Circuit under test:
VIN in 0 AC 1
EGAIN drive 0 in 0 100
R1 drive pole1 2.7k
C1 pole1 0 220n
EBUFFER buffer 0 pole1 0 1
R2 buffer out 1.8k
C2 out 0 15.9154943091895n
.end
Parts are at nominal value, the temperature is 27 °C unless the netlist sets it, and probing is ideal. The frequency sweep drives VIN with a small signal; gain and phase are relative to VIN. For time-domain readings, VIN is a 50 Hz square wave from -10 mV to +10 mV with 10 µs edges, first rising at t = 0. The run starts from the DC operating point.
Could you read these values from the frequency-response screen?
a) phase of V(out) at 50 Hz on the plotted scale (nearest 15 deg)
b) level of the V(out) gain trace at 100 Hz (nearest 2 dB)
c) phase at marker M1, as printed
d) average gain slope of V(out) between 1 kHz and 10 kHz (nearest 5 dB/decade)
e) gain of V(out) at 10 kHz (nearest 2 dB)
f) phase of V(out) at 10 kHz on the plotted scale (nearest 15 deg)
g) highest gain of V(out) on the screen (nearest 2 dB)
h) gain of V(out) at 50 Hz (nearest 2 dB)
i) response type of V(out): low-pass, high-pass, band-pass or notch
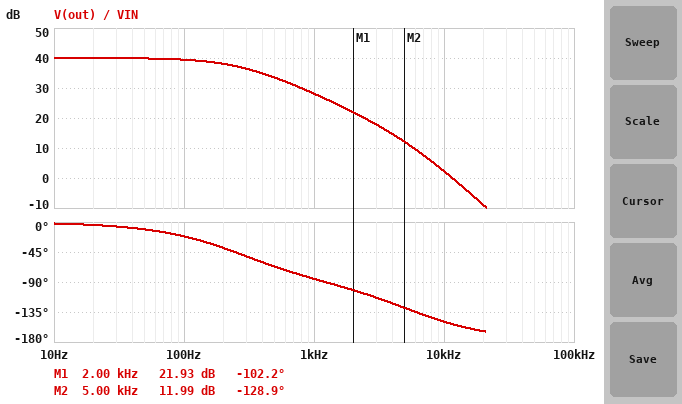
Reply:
-15 deg
40 dB
-102.2 deg
-25 dB/decade
2 dB
-150 deg
40 dB
40 dB
low-pass
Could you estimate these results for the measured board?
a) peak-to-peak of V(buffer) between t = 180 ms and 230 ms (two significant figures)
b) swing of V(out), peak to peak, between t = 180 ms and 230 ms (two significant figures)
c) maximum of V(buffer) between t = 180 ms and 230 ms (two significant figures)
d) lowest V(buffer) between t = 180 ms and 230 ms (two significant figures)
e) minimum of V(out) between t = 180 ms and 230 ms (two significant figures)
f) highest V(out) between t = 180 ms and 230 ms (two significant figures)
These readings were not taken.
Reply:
2.0 V
2.0 V
1.0 V
-1.0 V
-1.0 V
1.0 V
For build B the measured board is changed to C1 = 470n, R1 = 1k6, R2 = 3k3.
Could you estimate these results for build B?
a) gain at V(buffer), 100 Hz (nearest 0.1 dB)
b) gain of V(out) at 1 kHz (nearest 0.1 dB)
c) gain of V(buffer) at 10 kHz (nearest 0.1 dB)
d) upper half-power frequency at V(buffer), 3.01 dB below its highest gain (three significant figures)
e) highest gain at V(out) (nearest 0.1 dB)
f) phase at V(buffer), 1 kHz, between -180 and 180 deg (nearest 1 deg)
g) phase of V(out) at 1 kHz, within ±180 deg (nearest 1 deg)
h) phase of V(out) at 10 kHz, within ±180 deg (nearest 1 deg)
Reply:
39.1 dB
25.9 dB
6.5 dB
212 Hz
40.0 dB
-78 deg
-96 deg
-162 deg
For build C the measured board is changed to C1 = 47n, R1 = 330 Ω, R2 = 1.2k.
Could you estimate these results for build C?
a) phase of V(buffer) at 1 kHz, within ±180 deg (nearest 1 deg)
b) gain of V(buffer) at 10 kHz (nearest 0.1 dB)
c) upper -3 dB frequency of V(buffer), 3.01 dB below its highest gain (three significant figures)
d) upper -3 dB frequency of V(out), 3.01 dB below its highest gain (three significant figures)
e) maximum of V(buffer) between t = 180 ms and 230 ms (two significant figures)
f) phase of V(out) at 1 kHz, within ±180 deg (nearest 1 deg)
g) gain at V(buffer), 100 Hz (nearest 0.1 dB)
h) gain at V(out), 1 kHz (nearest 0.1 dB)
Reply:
-6 deg
37.1 dB
10.3 kHz
5.91 kHz
1.0 V
-12 deg
40.0 dB
39.9 dB
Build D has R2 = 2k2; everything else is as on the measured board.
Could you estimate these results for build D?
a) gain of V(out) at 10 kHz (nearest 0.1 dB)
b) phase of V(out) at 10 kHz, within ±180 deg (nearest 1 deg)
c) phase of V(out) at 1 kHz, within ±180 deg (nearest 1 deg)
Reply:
0.9 dB
-154 deg
-87 deg
